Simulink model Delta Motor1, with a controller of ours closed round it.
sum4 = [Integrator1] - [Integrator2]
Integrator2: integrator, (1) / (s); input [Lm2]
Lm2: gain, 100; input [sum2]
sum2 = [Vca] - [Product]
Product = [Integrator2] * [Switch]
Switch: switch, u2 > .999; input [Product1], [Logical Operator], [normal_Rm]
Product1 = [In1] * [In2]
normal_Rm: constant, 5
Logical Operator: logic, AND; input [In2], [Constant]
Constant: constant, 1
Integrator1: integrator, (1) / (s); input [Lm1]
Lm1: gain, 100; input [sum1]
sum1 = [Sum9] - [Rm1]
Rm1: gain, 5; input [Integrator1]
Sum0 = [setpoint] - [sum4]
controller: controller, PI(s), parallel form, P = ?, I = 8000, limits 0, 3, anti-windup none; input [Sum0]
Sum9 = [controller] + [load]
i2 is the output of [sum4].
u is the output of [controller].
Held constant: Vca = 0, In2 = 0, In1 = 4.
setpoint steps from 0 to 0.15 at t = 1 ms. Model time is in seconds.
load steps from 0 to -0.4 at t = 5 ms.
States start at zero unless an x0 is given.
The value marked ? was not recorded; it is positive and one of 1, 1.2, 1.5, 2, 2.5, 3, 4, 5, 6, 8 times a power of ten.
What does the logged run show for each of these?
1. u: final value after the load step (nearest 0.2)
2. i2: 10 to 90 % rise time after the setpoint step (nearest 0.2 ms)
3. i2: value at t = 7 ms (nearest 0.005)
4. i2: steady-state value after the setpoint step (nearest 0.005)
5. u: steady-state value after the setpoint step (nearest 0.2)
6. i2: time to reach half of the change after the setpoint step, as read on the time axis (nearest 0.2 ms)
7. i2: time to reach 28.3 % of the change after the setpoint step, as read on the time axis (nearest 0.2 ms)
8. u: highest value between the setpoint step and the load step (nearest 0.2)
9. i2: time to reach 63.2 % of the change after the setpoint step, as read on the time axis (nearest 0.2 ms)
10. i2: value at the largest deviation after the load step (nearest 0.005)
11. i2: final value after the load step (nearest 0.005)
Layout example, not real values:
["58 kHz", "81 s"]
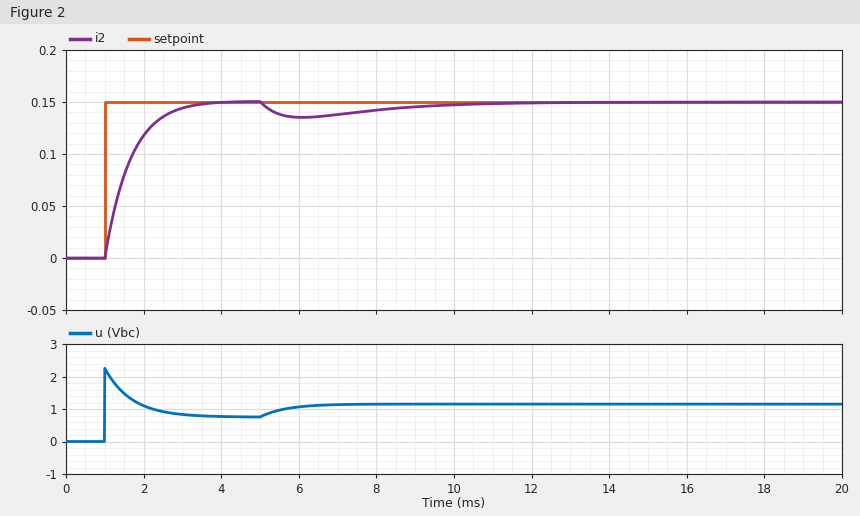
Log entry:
["1.2", "1.4 ms", "0.140", "0.150", "0.8", "1.4 ms", "1.2 ms", "2.2", "1.6 ms", "0.135", "0.150"]
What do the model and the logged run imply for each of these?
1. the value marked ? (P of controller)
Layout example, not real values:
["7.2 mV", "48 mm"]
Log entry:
["15"]
